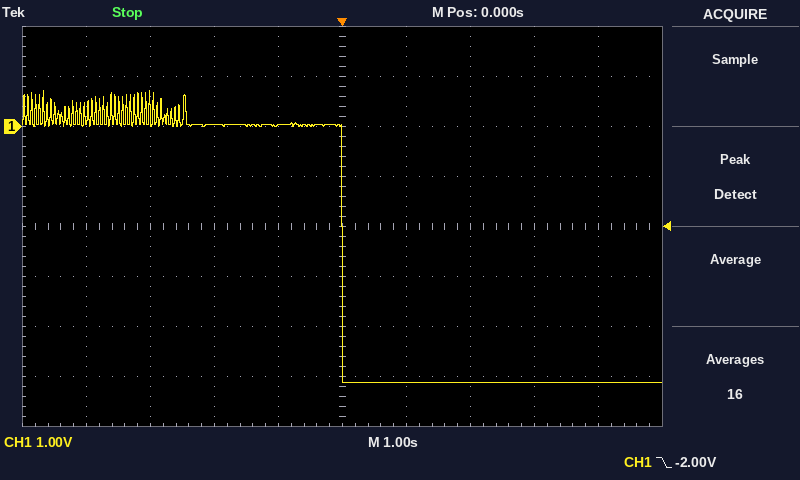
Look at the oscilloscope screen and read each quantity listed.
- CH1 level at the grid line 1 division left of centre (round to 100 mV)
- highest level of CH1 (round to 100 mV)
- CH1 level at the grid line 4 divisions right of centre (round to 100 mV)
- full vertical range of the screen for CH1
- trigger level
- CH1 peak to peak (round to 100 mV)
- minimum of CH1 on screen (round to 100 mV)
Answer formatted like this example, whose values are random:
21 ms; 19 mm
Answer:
0.0 V; 700 mV; -5.1 V; 8 V; -2.00 V; 5.8 V; -5.1 V
